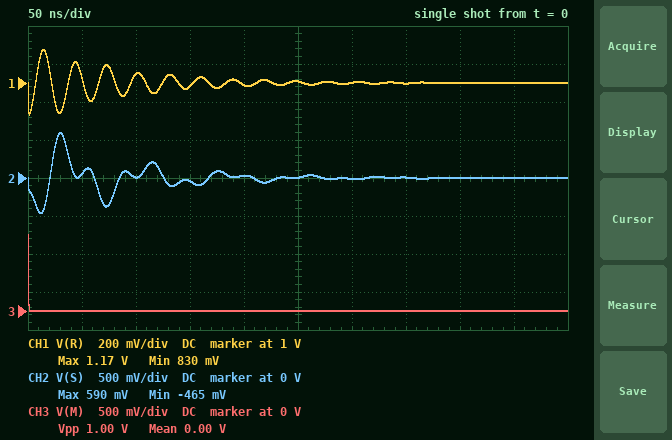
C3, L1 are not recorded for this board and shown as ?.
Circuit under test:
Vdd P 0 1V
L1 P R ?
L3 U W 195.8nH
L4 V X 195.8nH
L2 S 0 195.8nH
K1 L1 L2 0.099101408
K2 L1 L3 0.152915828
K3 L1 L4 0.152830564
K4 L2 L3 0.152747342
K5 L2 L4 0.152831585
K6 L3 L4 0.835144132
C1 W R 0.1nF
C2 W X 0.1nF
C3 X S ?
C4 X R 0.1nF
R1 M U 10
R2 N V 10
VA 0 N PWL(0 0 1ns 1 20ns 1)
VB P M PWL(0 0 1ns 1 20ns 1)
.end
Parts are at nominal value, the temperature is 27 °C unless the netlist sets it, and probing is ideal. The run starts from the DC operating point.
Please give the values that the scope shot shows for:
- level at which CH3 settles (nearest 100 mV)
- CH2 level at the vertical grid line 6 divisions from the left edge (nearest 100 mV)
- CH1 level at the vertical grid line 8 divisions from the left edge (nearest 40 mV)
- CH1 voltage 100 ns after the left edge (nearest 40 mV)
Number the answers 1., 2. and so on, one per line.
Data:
1. 0 V
2. 0 V
3. 1.00 V
4. 1.04 V
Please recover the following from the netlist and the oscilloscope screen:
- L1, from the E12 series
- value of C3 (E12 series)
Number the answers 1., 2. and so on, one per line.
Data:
1. 56 nH
2. 270 pF
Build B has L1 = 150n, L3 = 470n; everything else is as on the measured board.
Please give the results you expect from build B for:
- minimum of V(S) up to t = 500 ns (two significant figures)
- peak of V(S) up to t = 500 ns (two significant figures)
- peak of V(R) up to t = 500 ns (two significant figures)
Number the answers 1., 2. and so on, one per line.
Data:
1. -300 mV
2. 380 mV
3. 1.1 V
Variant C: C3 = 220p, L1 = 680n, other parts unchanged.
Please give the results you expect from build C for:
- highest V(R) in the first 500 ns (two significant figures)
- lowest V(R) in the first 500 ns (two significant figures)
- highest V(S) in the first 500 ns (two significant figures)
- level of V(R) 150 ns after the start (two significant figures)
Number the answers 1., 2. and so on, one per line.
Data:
1. 1.7 V
2. 230 mV
3. 280 mV
4. 520 mV
